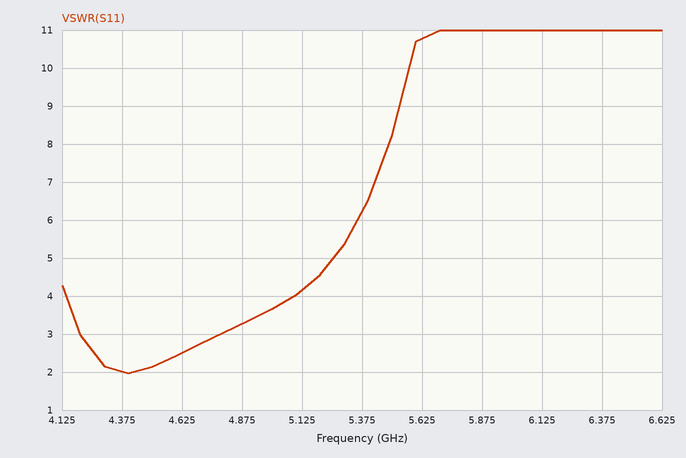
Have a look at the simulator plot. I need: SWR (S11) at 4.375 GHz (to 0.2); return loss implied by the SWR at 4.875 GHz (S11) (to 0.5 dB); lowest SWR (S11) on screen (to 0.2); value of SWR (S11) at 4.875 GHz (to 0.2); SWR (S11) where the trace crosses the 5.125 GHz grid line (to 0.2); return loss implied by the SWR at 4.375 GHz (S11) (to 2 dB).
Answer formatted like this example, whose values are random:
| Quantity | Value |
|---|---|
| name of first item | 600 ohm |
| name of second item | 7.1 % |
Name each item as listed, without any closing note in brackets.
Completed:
| Quantity | Value |
|---|---|
| SWR (S11) at 4.375 GHz | 2.0 |
| return loss implied by the SWR at 4.875 GHz (S11) | 5.5 dB |
| lowest SWR (S11) on screen | 2.0 |
| value of SWR (S11) at 4.875 GHz | 3.2 |
| SWR (S11) where the trace crosses the 5.125 GHz grid line | 4.2 |
| return loss implied by the SWR at 4.375 GHz (S11) | 10 dB |
